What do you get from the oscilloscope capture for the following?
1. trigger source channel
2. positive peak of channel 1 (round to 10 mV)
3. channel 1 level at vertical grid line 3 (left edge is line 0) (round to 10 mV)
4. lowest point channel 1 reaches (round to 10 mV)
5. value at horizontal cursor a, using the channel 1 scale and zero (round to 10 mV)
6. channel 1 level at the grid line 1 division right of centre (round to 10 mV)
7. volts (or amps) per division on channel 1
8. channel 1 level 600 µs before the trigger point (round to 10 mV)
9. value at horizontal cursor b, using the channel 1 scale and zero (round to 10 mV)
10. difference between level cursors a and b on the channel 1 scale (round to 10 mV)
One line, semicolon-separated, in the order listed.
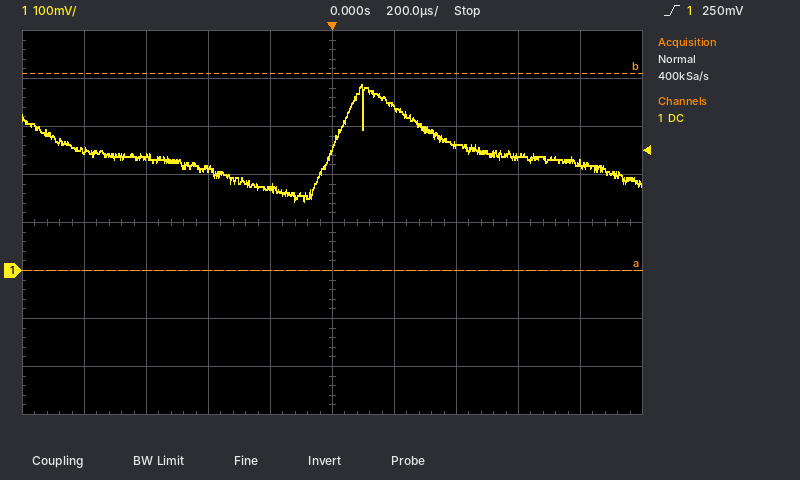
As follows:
channel 1; 390 mV; 210 mV; 140 mV; 0 mV; 340 mV; 100 mV; 240 mV; 410 mV; 410 mV
